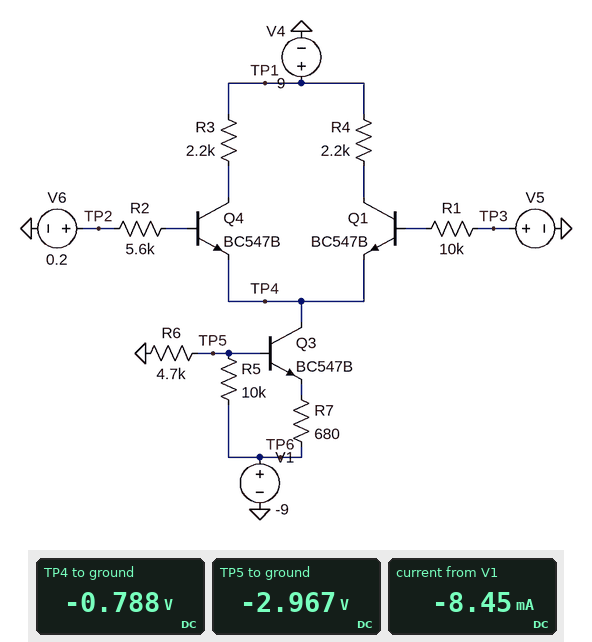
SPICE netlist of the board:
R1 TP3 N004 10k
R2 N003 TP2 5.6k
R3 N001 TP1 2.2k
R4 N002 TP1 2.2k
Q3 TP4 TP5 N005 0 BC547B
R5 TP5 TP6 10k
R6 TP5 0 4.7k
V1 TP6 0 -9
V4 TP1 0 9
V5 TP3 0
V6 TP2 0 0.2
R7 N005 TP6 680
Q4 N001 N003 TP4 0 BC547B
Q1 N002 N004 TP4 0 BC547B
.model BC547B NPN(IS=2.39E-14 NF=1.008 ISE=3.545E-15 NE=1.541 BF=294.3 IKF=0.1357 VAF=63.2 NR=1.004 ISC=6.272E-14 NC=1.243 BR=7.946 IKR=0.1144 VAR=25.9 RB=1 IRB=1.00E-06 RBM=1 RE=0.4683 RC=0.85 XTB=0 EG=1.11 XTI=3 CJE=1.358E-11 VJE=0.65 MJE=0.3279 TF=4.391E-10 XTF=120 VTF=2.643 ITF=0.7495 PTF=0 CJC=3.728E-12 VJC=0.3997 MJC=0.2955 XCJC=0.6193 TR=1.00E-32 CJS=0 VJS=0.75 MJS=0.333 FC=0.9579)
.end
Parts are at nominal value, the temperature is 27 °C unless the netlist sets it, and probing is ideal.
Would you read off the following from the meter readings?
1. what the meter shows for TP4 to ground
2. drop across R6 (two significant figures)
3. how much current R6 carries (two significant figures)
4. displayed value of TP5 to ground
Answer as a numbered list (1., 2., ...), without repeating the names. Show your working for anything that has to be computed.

1. -0.788 V
2. 0 V - (-2.967 V) = 3.0 V
3. (0 V - (-2.967 V)) / 4.7 kΩ = 630 µA
4. -2.967 V
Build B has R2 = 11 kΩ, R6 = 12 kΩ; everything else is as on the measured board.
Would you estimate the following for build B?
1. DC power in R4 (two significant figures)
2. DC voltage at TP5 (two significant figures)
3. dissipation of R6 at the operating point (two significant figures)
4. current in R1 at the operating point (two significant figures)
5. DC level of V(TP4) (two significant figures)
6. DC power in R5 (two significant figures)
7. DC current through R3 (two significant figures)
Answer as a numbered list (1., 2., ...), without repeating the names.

1. 970 µW
2. -5.0 V
3. 2.1 mW
4. 2.1 µA
5. -650 mV
6. 1.6 mW
7. 4.2 mA
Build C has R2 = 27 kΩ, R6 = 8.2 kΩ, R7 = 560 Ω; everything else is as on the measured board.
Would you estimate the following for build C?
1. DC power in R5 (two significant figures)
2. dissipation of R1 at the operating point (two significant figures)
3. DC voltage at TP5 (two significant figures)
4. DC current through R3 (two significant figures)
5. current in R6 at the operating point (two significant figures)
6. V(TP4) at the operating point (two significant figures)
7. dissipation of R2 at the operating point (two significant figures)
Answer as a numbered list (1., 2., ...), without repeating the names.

1. 2.3 mW
2. 1.8 µW
3. -4.2 V
4. 3.5 mA
5. 510 µA
6. -810 mV
7. 4.2 µW
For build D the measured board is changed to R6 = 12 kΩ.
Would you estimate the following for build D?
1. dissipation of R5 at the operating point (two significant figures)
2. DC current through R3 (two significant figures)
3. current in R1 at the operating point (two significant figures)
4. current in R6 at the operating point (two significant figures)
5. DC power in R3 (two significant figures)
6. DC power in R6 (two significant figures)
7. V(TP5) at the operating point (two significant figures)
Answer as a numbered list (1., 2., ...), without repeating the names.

1. 1.6 mW
2. 4.3 mA
3. 1.6 µA
4. 420 µA
5. 41 mW
6. 2.1 mW
7. -5.0 V
